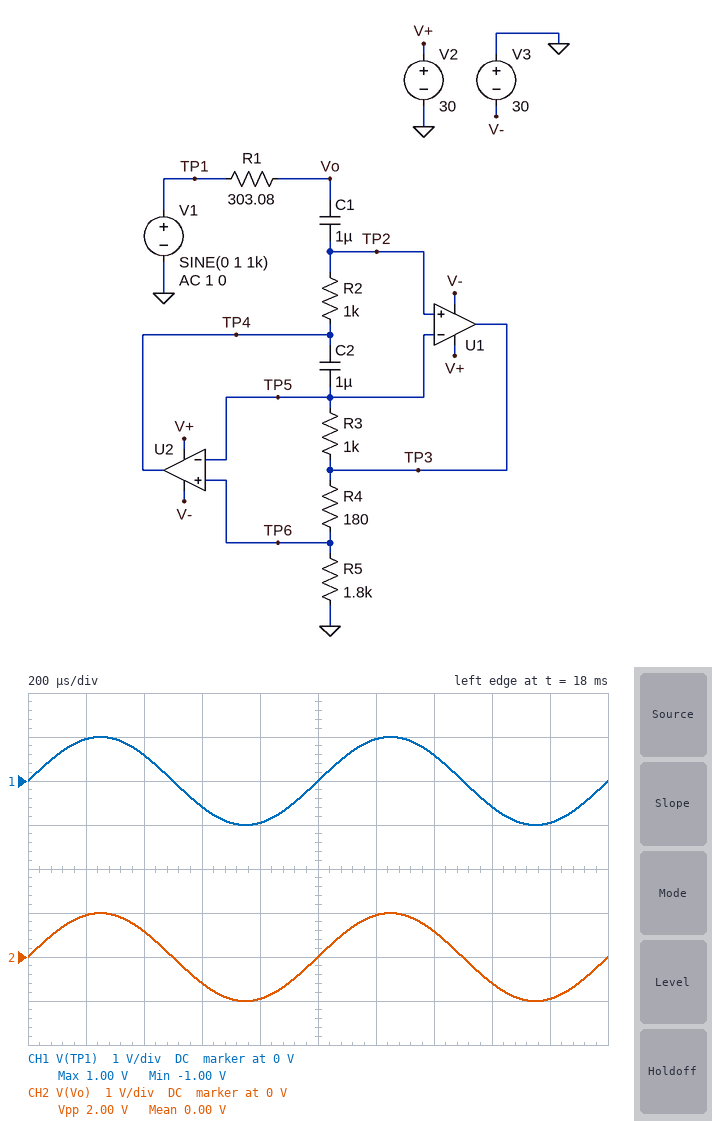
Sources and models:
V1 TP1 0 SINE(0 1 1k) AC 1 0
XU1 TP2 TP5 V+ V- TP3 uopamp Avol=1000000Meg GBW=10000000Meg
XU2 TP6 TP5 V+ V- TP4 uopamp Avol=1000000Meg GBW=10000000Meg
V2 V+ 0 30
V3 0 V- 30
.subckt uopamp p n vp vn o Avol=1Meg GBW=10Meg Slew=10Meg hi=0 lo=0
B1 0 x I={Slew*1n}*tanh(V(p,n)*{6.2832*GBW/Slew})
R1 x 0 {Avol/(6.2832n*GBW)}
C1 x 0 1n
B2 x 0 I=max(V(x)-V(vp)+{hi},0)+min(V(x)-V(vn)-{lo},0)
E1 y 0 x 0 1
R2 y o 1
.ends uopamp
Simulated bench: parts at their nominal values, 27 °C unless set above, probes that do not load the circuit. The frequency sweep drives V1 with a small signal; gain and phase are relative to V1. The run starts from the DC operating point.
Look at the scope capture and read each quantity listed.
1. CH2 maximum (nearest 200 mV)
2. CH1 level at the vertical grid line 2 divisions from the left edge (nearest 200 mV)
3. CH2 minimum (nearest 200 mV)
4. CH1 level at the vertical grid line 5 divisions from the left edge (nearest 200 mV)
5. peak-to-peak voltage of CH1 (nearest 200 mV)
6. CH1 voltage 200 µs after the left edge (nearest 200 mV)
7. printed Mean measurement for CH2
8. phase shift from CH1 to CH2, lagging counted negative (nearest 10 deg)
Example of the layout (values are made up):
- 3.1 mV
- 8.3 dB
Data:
- 1.0 V
- 600 mV
- -1.0 V
- 0 V
- 2.0 V
- 1.0 V
- 0.00 V
- 0 deg
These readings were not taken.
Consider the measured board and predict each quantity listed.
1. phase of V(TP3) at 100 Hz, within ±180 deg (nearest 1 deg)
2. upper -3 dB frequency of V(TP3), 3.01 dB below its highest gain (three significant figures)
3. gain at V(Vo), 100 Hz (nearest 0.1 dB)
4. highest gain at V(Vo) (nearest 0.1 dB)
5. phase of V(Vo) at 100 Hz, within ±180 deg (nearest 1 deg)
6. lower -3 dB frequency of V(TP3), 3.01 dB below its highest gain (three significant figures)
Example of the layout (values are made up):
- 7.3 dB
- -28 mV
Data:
- 4 deg
- 53.1 Hz
- 0 dB
- 0 dB
- 4 deg
- 48.2 Hz
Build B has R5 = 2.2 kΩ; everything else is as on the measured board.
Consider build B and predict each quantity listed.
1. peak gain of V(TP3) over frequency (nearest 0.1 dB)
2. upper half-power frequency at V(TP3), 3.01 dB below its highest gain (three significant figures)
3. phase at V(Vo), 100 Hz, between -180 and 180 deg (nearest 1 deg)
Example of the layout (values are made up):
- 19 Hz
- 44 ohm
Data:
- 21.9 dB
- 47.7 Hz
- 3 deg
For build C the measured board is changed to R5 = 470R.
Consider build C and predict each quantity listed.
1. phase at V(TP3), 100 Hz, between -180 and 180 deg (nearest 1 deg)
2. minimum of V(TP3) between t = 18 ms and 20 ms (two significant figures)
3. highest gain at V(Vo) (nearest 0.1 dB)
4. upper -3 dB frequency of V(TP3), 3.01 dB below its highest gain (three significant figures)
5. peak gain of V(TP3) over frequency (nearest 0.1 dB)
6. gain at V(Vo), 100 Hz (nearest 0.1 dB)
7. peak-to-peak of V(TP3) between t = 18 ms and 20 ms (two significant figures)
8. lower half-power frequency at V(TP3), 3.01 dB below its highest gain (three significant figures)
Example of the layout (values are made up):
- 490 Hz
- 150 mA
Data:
- 81 deg
- -1.4 V
- 0 dB
- 110 Hz
- 17.4 dB
- -15.9 dB
- 2.8 V
- 91.1 Hz
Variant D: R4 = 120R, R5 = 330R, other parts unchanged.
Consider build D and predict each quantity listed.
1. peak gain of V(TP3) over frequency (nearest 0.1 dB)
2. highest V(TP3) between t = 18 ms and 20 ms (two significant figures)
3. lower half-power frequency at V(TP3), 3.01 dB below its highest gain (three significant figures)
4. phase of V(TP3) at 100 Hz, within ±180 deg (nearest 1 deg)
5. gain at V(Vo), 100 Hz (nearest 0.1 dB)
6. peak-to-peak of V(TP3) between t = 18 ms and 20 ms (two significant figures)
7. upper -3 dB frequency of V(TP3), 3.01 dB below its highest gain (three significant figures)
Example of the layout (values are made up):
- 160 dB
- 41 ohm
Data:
- 17.5 dB
- 1.4 V
- 88.9 Hz
- 66 deg
- -7.7 dB
- 2.8 V
- 107 Hz
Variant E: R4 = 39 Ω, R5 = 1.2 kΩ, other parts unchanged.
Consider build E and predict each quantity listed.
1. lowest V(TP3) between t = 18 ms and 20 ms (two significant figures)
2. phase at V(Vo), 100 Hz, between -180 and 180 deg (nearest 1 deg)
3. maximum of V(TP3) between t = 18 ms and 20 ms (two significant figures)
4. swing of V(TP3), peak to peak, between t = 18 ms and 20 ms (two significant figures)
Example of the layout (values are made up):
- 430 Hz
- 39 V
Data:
- -1.0 V
- 1 deg
- 1.0 V
- 2.1 V
